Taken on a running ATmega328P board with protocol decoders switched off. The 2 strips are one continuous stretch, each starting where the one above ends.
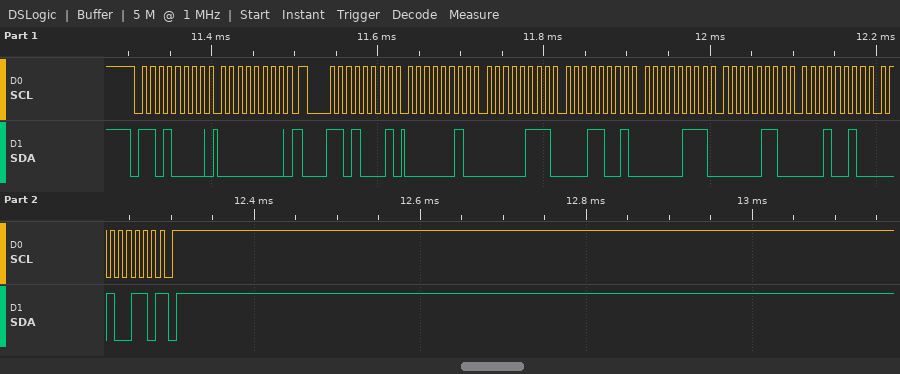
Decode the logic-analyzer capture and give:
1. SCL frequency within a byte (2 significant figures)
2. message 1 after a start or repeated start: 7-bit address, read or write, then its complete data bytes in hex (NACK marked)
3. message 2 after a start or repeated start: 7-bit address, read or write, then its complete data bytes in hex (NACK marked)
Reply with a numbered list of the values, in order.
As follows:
1. 100 kHz
2. 0x68 write: 00
3. 0x68 read: 02 07 19 07 06 12 26 NACK
